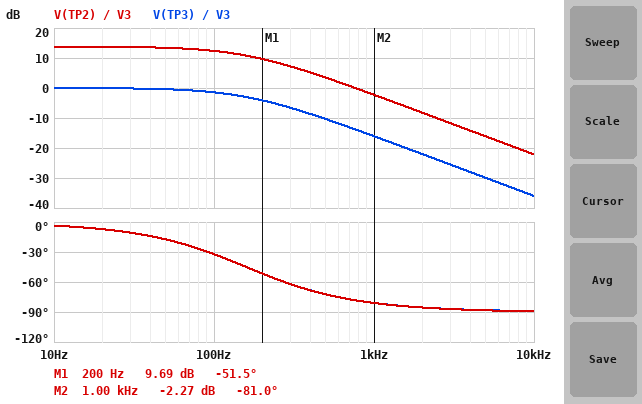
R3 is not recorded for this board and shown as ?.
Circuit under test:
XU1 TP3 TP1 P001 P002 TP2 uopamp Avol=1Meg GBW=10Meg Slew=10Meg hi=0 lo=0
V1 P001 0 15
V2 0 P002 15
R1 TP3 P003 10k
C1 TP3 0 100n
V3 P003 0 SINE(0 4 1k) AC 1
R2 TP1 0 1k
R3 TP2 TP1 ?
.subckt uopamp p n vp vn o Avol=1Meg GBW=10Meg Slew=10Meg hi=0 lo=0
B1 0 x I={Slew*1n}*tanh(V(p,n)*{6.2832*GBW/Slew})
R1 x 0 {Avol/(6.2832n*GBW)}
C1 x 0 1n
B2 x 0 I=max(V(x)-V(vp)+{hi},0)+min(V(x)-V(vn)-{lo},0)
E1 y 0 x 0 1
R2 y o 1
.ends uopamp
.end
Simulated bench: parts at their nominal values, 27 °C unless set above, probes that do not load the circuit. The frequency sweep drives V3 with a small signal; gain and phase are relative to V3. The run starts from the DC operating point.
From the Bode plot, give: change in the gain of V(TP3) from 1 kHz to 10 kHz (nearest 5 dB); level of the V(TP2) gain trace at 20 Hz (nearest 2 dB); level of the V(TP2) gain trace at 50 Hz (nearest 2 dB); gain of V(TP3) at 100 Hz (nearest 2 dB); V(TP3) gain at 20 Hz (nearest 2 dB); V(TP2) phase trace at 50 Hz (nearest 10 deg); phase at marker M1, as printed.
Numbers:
-20 dB
14 dB
14 dB
-2 dB
0 dB
-20 deg
-51.5 deg
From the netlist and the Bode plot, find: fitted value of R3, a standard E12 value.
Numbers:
3.9 kΩ
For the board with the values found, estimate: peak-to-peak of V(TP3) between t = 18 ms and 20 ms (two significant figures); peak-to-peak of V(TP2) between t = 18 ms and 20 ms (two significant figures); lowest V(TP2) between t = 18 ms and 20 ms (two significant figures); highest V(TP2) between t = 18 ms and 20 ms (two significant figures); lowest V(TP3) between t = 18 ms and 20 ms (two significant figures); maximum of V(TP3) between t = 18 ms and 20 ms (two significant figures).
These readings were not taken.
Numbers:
1.3 V
6.2 V
-3.1 V
3.1 V
-630 mV
630 mV
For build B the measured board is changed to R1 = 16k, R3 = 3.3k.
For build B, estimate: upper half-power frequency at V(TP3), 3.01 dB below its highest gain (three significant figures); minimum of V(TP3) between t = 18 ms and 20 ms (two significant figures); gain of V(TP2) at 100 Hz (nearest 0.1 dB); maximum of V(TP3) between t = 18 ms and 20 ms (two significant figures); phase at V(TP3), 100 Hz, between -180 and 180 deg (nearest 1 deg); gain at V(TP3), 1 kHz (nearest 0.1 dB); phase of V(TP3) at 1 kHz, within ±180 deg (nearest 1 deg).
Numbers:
99.5 Hz
-400 mV
9.6 dB
400 mV
-45 deg
-20.1 dB
-84 deg
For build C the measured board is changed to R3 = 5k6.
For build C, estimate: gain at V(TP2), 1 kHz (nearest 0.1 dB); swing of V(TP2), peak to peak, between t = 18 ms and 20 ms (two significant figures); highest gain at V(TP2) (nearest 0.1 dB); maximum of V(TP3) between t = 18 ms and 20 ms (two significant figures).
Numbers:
0.3 dB
8.3 V
16.4 dB
630 mV
